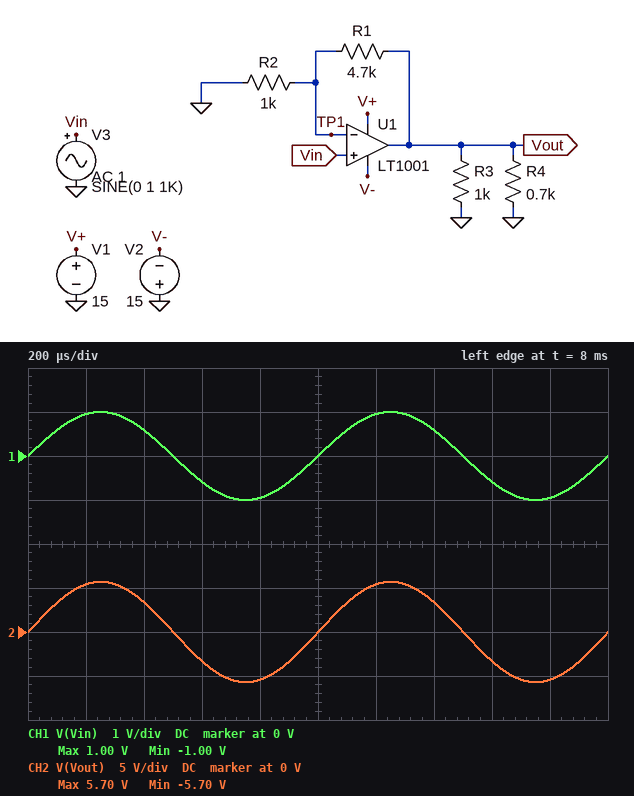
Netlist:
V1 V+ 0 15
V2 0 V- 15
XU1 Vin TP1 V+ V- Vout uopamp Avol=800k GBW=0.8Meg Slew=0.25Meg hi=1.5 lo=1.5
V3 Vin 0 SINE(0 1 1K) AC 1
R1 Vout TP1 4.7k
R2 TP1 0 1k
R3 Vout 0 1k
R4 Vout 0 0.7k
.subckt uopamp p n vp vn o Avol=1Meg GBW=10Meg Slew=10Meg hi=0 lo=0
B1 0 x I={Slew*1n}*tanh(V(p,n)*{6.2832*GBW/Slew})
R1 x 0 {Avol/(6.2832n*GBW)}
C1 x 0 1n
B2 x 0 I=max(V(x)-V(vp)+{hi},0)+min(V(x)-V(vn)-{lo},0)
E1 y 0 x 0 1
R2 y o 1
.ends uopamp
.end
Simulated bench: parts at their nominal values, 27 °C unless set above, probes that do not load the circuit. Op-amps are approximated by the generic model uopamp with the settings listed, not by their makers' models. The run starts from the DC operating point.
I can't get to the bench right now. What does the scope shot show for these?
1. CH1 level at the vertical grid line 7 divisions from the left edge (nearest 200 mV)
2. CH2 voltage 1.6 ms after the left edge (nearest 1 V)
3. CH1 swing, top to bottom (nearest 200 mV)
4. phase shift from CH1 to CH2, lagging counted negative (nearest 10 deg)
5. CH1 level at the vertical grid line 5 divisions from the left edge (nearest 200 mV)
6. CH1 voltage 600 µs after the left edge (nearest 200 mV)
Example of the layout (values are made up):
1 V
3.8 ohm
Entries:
600 mV
-3 V
2.0 V
0 deg
0 V
-600 mV
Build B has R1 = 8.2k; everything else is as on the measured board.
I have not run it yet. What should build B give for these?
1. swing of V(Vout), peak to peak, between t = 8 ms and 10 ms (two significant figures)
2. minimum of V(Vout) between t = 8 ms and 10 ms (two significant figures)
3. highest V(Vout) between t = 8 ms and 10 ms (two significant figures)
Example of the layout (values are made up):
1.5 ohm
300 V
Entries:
18 V
-9.2 V
9.2 V
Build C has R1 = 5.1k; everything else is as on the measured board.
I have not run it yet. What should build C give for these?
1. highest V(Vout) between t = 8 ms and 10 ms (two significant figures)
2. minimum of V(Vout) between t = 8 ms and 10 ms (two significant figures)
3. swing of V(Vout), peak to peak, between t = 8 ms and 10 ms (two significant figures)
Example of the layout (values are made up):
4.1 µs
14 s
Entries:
6.1 V
-6.1 V
12 V
